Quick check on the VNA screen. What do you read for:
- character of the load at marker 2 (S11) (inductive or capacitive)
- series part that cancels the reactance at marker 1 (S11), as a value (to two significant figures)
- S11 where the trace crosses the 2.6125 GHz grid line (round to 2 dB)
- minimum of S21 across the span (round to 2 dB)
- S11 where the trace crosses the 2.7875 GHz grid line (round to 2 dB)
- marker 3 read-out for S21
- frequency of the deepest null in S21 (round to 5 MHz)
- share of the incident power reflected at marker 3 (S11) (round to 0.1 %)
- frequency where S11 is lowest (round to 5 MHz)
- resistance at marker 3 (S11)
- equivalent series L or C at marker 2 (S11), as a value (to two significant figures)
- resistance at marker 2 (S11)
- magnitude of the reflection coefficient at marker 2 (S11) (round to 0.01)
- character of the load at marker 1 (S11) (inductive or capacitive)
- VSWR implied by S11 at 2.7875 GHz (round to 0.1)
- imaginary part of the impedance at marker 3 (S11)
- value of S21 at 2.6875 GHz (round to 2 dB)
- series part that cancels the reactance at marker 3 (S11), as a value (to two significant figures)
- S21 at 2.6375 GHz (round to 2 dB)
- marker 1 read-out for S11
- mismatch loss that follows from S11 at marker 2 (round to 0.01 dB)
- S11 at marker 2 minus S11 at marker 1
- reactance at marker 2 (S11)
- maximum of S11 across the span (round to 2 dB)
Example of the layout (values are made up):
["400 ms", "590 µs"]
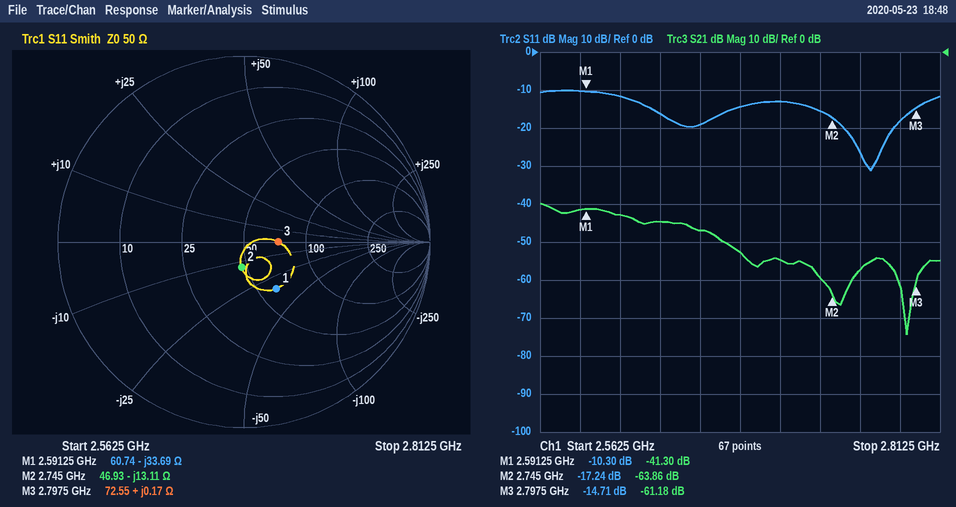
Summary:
["capacitive", "2.1 nH", "-12 dB", "-74 dB", "-18 dB", "-61.18 dB", "2.790 GHz", "3.4 %", "2.770 GHz", "72.55 Ω", "4.4 pF", "46.93 Ω", "0.14", "capacitive", "1.3", "+0.17 Ω", "-52 dB", "330 pF", "-44 dB", "-10.30 dB", "0.08 dB", "-6.94 dB", "-13.11 Ω", "-10 dB"]
